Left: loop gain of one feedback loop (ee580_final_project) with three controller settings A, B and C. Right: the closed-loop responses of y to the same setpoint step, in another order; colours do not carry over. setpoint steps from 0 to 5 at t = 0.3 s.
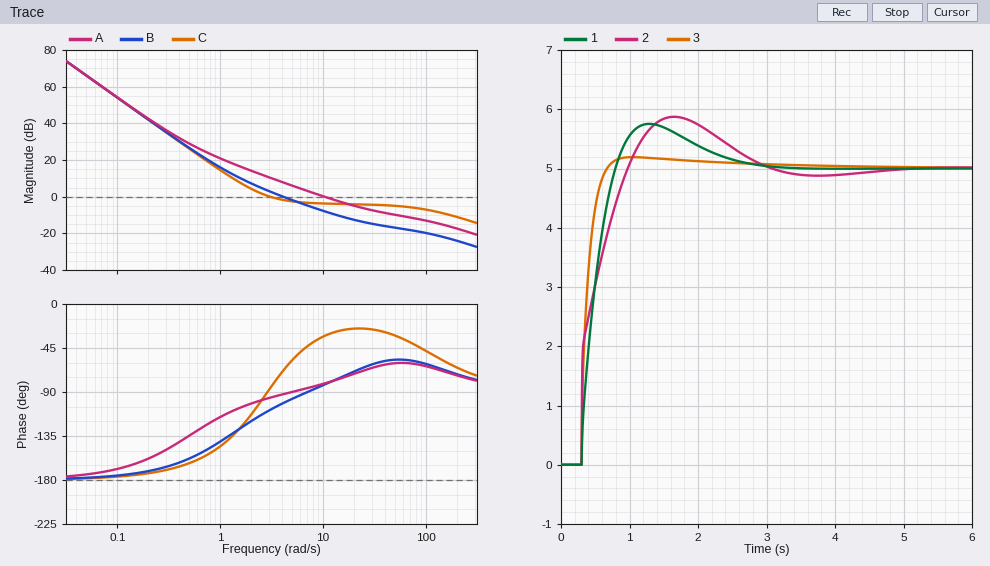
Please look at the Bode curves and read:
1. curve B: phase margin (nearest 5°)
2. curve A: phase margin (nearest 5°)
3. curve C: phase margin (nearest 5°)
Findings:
80°
100°
95°
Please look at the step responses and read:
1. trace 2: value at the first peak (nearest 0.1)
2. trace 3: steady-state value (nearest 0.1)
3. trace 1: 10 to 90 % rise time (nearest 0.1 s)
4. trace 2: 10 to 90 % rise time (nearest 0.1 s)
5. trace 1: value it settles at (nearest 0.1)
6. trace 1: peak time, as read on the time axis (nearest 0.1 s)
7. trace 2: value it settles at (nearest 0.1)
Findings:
5.9
5.0
0.4 s
0.5 s
5.0
1.3 s
5.0
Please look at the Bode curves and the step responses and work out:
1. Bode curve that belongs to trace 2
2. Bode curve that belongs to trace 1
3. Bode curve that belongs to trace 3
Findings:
C
B
A
